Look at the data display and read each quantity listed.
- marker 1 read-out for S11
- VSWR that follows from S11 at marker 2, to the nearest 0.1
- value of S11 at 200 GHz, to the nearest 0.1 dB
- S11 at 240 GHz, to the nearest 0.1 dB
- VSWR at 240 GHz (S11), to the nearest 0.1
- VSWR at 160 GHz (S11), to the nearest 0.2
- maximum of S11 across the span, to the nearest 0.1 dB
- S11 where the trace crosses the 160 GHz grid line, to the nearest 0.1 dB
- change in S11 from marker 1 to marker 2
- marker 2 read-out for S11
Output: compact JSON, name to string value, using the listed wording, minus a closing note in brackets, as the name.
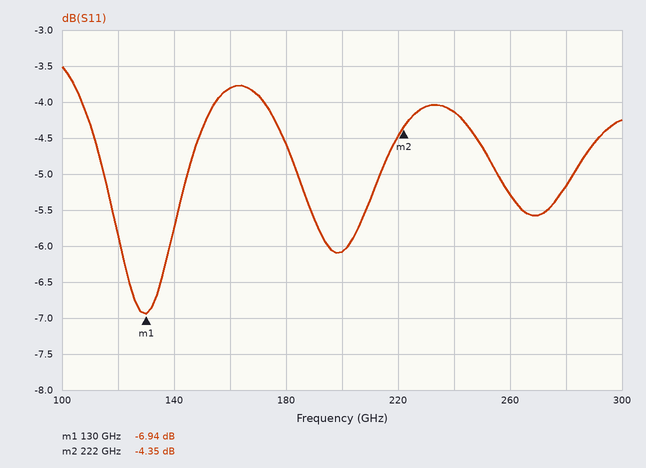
{"marker 1 read-out for S11": "-6.94 dB", "VSWR that follows from S11 at marker 2, to the nearest 0.1": "4.1", "value of S11 at 200 GHz, to the nearest 0.1 dB": "-6.1 dB", "S11 at 240 GHz, to the nearest 0.1 dB": "-4.1 dB", "VSWR at 240 GHz (S11), to the nearest 0.1": "4.3", "VSWR at 160 GHz (S11), to the nearest 0.2": "4.6", "maximum of S11 across the span, to the nearest 0.1 dB": "-3.5 dB", "S11 where the trace crosses the 160 GHz grid line, to the nearest 0.1 dB": "-3.8 dB", "change in S11 from marker 1 to marker 2": "2.59 dB", "marker 2 read-out for S11": "-4.35 dB"}
